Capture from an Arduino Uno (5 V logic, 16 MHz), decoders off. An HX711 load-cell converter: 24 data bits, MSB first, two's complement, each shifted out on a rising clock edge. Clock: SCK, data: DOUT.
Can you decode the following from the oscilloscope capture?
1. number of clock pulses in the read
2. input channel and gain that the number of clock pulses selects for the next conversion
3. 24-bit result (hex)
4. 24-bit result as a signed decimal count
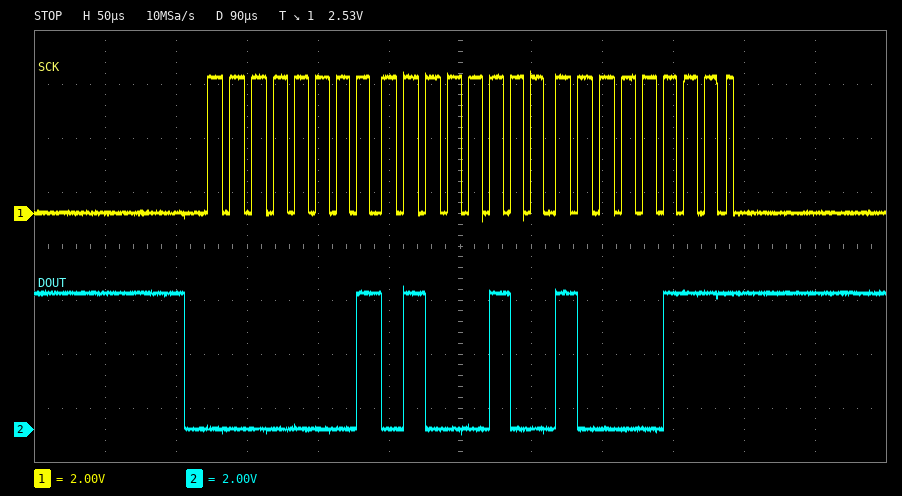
25
channel A, gain 128
0x014487
83079
